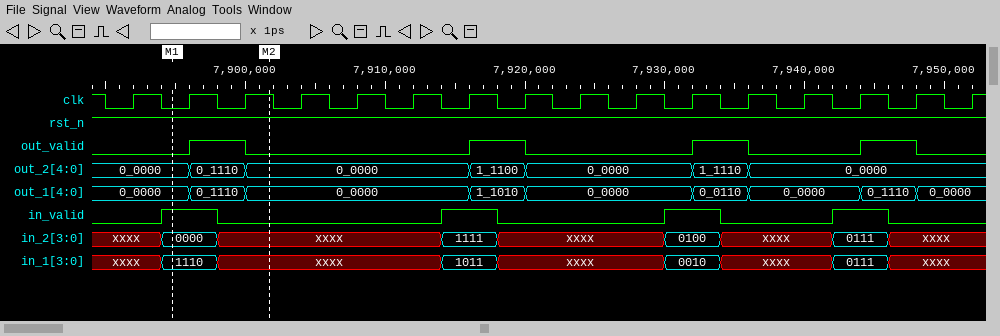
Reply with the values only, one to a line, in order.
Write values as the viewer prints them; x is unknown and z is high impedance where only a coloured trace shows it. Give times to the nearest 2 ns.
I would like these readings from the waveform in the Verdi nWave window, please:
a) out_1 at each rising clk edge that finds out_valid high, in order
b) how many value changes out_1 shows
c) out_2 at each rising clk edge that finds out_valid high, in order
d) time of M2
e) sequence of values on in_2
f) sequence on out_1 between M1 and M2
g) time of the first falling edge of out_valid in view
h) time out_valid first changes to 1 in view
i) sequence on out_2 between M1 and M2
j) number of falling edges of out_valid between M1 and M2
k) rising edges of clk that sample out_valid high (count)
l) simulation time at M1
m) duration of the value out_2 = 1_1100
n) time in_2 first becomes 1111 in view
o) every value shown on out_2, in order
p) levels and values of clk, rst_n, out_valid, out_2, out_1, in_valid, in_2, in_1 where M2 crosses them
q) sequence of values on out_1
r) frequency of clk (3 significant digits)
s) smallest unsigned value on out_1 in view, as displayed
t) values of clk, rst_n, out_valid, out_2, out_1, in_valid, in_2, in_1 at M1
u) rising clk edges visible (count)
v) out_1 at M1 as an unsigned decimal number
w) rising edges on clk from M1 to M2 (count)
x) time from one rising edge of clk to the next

0_1110, 1_1010, 0_0110, 0_1110
8
0_1110, 1_1100, 1_1110, 0_0000
7902 ns
xxxx, 0000, xxxx, 1111, xxxx, 0100, xxxx, 0111, xxxx
0_0000, 0_1110, 0_0000
7900 ns
7896 ns
0_0000, 0_1110, 0_0000
1
4
7894 ns
4 ns
7914 ns
0_0000, 0_1110, 0_0000, 1_1100, 0_0000, 1_1110, 0_0000
clk=1, rst_n=1, out_valid=0, out_2=0_0000, out_1=0_0000, in_valid=0, in_2=xxxx, in_1=xxxx
0_0000, 0_1110, 0_0000, 1_1010, 0_0000, 0_0110, 0_0000, 0_1110, 0_0000
250 MHz
0_0000
clk=0, rst_n=1, out_valid=0, out_2=0_0000, out_1=0_0000, in_valid=1, in_2=0000, in_1=1110
16
0
2
4 ns
